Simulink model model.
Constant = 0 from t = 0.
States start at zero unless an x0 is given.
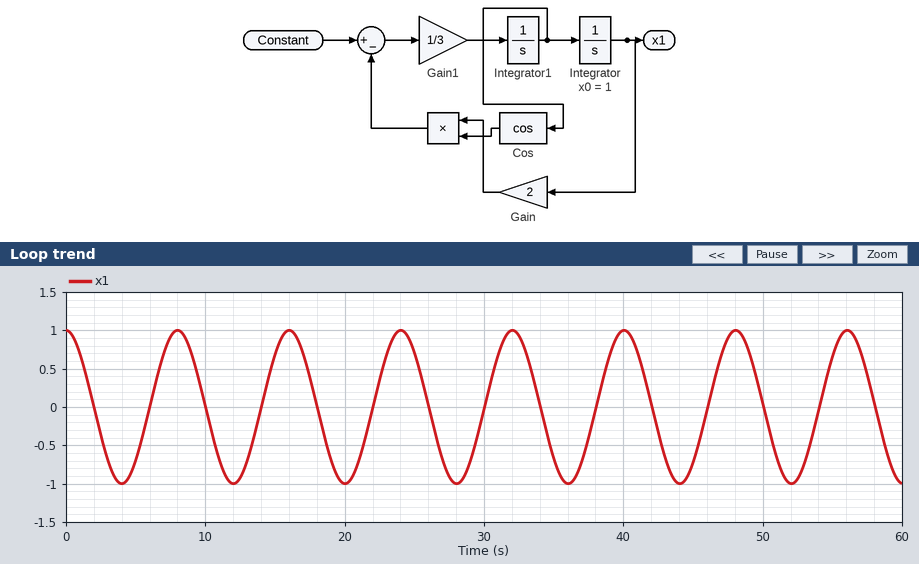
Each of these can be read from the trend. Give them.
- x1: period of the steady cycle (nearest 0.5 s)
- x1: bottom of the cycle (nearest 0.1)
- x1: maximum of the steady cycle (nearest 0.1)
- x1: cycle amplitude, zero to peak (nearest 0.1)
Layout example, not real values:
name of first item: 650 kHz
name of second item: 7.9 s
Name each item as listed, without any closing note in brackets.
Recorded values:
x1: period of the steady cycle: 8.0 s
x1: bottom of the cycle: -1.0
x1: maximum of the steady cycle: 1.0
x1: cycle amplitude, zero to peak: 1.0
